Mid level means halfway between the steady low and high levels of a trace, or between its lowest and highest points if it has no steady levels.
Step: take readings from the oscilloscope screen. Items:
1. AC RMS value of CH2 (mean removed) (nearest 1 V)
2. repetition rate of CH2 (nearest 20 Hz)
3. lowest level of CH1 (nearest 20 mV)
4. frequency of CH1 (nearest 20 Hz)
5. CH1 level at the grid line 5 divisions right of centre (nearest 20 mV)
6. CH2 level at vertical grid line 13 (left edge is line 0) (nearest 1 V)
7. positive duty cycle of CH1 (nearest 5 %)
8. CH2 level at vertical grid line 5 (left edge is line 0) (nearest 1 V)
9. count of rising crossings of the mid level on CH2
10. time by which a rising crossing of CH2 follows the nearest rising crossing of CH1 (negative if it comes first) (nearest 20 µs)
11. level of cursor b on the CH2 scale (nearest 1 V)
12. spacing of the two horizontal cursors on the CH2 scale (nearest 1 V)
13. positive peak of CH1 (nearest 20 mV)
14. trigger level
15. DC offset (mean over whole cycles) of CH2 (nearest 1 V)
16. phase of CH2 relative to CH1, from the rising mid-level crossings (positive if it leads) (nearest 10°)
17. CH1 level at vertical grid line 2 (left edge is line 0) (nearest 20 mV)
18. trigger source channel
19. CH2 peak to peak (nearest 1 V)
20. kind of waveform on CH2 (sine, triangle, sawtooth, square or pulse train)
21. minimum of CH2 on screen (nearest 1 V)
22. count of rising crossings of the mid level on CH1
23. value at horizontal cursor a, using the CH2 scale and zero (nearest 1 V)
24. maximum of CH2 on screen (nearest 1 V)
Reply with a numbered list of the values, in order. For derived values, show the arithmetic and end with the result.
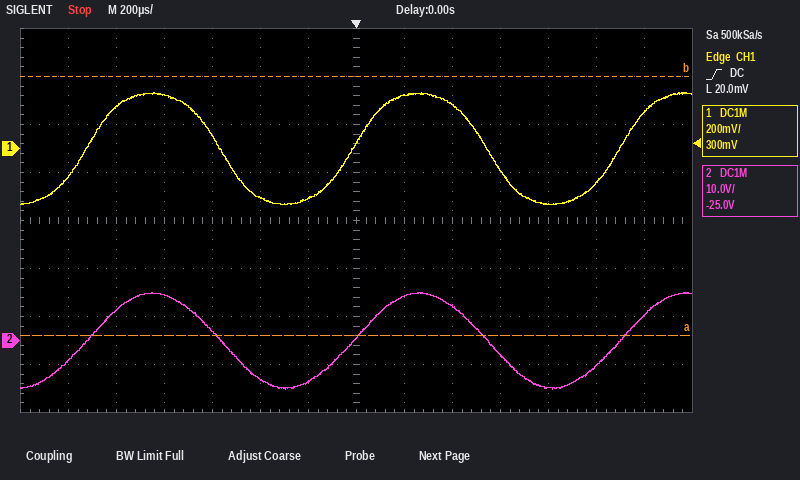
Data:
1. 20 V / (2√2) ≈ 7 V
2. 900 Hz
3. -240 mV
4. 900 Hz
5. -140 mV
6. 5 V
7. 50 %
8. -8 V
9. 3
10. 0 µs
11. 55 V
12. 54 V
13. 240 mV
14. 20.0 mV
15. (10 V + (-10 V)) / 2 ≈ 0 V
16. 0°
17. 180 mV
18. CH1
19. 10 V − (-10 V) = 20 V
20. sine
21. -10 V
22. 3
23. 1 V
24. 10 V
